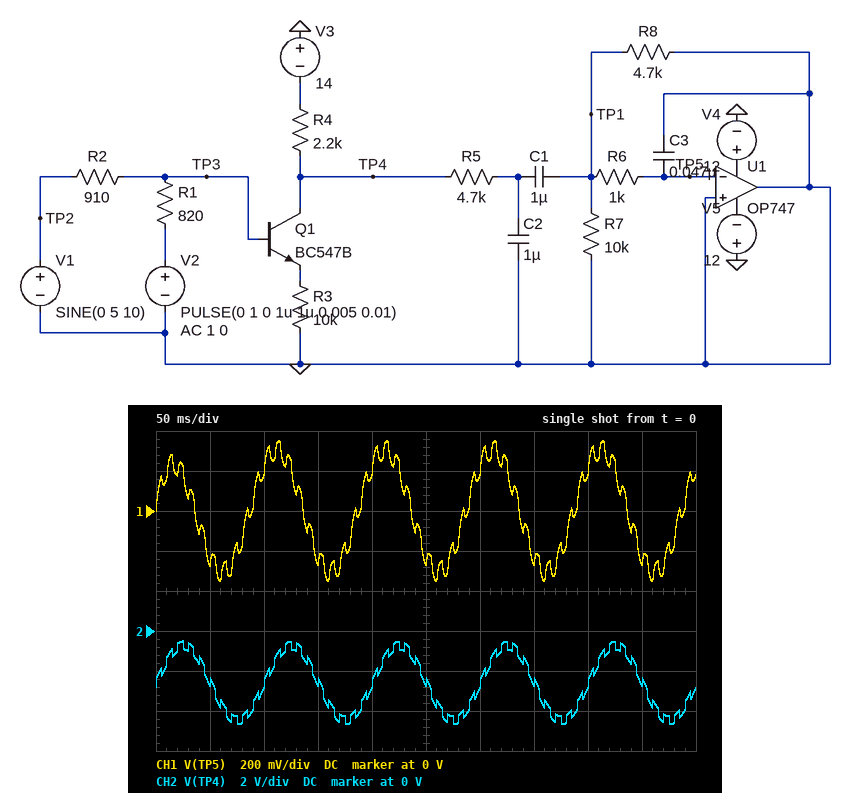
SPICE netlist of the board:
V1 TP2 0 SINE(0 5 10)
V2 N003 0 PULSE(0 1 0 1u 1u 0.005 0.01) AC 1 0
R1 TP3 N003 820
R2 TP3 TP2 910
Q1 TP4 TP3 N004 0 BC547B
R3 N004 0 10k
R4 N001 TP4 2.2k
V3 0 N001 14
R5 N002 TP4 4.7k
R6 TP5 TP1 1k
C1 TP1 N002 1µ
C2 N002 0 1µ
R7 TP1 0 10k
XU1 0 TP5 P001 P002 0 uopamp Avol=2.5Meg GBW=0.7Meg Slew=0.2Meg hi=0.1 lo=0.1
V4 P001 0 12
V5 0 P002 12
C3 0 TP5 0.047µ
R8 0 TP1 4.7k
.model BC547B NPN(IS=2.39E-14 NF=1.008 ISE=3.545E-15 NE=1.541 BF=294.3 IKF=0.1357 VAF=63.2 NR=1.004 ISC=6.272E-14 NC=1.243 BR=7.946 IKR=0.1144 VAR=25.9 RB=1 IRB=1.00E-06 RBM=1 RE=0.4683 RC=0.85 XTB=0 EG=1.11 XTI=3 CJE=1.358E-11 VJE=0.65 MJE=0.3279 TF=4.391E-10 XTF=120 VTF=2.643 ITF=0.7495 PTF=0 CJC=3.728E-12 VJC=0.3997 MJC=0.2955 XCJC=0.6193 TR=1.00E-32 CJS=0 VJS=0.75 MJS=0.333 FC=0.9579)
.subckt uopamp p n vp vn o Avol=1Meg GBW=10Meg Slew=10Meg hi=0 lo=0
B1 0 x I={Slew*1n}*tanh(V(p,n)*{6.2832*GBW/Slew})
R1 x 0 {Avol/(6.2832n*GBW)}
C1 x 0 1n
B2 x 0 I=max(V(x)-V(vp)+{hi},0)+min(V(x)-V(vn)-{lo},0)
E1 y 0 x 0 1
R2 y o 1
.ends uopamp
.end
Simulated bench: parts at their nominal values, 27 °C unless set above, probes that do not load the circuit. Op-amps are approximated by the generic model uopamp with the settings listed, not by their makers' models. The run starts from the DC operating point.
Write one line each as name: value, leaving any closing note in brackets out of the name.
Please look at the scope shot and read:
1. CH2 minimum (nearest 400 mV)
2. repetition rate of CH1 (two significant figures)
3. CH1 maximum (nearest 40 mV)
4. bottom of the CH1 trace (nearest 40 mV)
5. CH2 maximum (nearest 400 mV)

CH2 minimum: -4.8 V
repetition rate of CH1: 10 Hz
CH1 maximum: 360 mV
bottom of the CH1 trace: -360 mV
CH2 maximum: -400 mV
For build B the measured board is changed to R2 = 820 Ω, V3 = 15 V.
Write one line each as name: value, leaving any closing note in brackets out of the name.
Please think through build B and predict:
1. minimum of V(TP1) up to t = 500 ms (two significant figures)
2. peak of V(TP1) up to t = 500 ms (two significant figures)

minimum of V(TP1) up to t = 500 ms: -370 mV
peak of V(TP1) up to t = 500 ms: 370 mV
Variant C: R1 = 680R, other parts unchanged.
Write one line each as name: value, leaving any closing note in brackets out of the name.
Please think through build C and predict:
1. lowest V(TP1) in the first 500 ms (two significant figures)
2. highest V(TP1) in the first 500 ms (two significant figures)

lowest V(TP1) in the first 500 ms: -330 mV
highest V(TP1) in the first 500 ms: 330 mV
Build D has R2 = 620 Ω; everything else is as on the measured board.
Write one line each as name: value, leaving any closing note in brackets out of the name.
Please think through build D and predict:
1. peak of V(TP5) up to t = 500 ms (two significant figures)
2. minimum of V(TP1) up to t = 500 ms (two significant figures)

peak of V(TP5) up to t = 500 ms: 420 mV
minimum of V(TP1) up to t = 500 ms: -420 mV
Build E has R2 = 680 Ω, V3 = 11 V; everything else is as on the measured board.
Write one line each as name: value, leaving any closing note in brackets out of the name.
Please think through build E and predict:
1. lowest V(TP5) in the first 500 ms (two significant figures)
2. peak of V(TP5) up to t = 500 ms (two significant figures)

lowest V(TP5) in the first 500 ms: -400 mV
peak of V(TP5) up to t = 500 ms: 400 mV
